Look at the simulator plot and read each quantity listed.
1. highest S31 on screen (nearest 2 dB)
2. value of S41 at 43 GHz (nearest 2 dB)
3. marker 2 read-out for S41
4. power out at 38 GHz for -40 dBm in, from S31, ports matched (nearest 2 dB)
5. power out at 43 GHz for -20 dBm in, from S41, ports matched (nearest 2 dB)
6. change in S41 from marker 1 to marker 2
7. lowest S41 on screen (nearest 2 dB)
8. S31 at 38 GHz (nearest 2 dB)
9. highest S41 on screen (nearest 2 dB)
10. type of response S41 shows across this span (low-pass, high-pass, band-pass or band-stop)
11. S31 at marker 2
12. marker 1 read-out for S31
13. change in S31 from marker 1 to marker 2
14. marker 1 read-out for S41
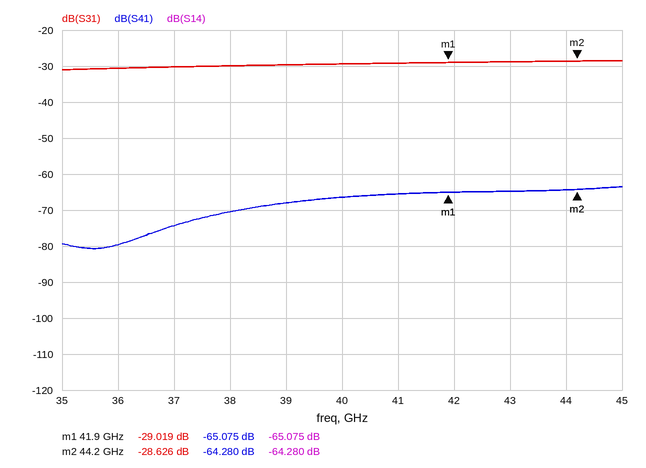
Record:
-28 dB
-64 dB
-64.280 dB
-70 dBm
-84 dBm
0.795 dB
-80 dB
-30 dB
-64 dB
high-pass
-28.626 dB
-29.019 dB
0.393 dB
-65.075 dB
